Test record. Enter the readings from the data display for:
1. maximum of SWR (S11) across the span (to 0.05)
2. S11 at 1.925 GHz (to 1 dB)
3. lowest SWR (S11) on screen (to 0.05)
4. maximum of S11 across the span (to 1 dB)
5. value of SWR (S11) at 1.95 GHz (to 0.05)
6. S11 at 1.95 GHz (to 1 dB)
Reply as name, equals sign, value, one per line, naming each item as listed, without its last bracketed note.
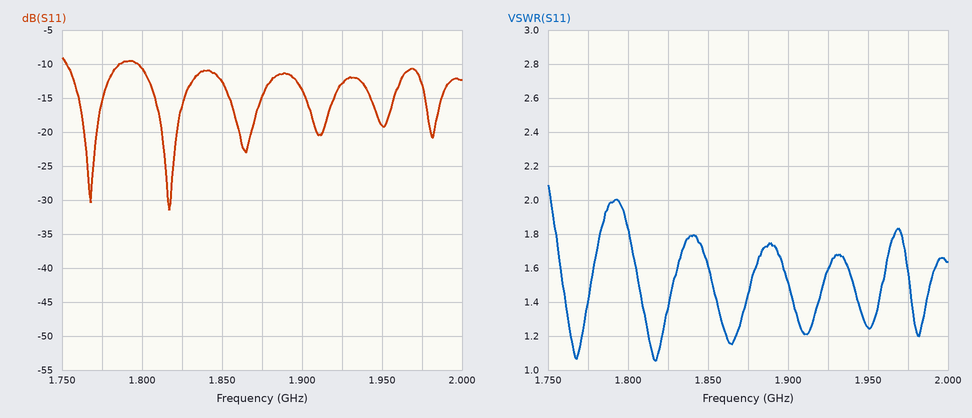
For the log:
maximum of SWR (S11) across the span = 2.10
S11 at 1.925 GHz = -13 dB
lowest SWR (S11) on screen = 1.05
maximum of S11 across the span = -9 dB
value of SWR (S11) at 1.95 GHz = 1.25
S11 at 1.95 GHz = -19 dB
